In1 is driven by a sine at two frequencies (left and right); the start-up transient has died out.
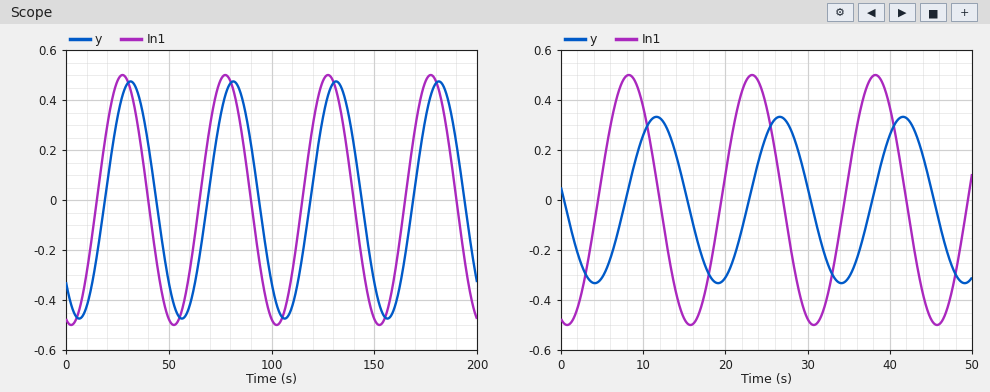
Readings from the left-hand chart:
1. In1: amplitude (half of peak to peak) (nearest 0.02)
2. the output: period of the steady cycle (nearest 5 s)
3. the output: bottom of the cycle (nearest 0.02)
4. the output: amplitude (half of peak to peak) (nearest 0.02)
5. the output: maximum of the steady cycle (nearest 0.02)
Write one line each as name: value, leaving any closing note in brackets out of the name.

In1: amplitude (half of peak to peak): 0.50
the output: period of the steady cycle: 50 s
the output: bottom of the cycle: -0.48
the output: amplitude (half of peak to peak): 0.48
the output: maximum of the steady cycle: 0.48
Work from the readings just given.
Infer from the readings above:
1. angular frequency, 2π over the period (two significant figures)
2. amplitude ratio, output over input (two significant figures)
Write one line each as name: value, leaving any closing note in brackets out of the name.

angular frequency, 2π over the period: 0.13 rad/s
amplitude ratio, output over input: 0.96
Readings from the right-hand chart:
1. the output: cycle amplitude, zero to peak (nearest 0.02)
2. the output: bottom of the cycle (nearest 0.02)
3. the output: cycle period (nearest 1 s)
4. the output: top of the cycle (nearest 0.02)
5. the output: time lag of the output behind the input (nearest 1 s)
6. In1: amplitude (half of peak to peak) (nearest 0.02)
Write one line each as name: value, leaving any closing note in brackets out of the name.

the output: cycle amplitude, zero to peak: 0.34
the output: bottom of the cycle: -0.34
the output: cycle period: 15 s
the output: top of the cycle: 0.34
the output: time lag of the output behind the input: 3 s
In1: amplitude (half of peak to peak): 0.50
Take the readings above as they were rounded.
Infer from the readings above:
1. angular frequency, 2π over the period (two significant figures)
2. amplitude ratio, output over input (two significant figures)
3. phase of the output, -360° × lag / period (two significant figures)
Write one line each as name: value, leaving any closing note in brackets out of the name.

angular frequency, 2π over the period: 0.42 rad/s
amplitude ratio, output over input: 0.68
phase of the output, -360° × lag / period: -72°
